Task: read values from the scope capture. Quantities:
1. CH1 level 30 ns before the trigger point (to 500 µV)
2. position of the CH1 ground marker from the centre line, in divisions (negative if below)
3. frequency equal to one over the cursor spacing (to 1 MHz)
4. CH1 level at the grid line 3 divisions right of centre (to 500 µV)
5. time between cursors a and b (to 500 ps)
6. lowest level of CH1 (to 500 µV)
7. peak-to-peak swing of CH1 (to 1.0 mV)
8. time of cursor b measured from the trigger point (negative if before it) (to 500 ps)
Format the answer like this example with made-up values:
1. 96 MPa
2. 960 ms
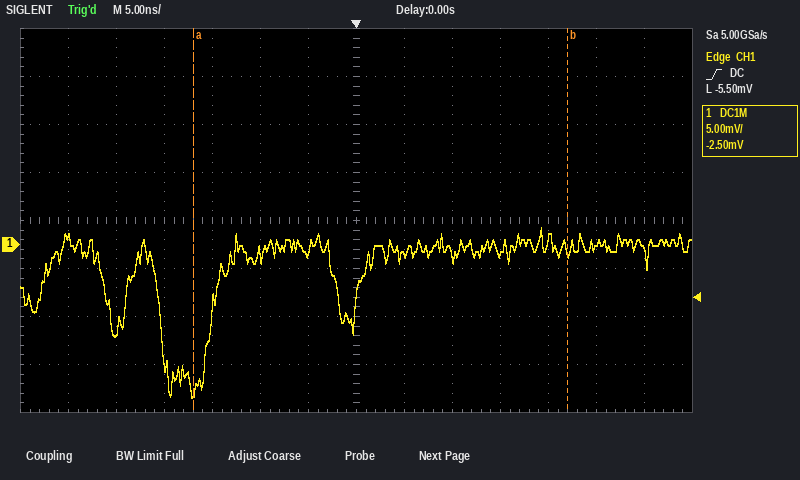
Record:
1. 1.0 mV
2. -0.5 div
3. 26 MHz
4. -1.0 mV
5. 39.0 ns
6. -16.0 mV
7. 18.0 mV
8. +22.0 ns
